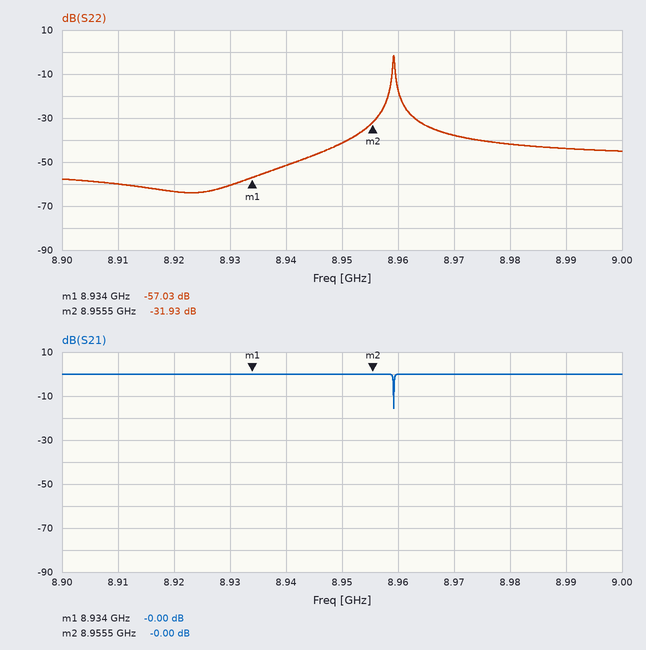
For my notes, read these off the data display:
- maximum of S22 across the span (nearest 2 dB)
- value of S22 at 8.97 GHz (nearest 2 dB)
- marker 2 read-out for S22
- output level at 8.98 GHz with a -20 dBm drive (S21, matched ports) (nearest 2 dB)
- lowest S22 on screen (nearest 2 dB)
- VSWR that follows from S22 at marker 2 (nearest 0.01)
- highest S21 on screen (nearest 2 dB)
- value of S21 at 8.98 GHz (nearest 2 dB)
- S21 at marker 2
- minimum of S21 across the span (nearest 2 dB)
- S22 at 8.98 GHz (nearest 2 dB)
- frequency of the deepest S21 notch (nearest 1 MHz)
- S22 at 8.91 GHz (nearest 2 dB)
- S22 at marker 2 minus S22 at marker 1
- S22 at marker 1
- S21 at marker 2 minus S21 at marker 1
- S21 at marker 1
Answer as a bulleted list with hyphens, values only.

- -2 dB
- -38 dB
- -31.93 dB
- -20 dBm
- -64 dB
- 1.05
- 0 dB
- 0 dB
- -0.00 dB
- -16 dB
- -42 dB
- 8.959 GHz
- -60 dB
- 25.10 dB
- -57.03 dB
- 0.00 dB
- -0.00 dB
